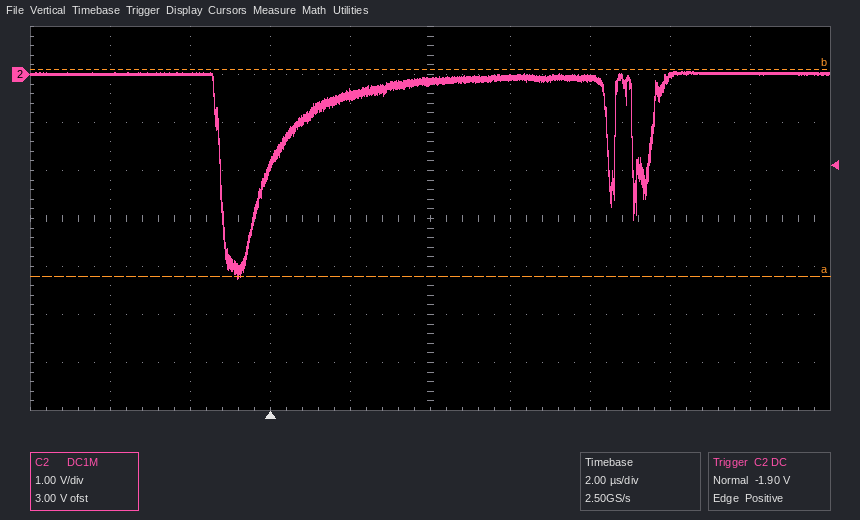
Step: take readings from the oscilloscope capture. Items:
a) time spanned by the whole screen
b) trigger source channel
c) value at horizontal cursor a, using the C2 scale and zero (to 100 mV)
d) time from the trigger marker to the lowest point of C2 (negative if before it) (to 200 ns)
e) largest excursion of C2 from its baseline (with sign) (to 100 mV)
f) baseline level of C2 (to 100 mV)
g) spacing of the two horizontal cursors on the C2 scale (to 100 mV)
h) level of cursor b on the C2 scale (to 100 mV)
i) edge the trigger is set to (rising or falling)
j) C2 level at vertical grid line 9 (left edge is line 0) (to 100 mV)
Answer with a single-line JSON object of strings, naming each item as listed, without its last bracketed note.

{"time spanned by the whole screen": "20 µs", "trigger source channel": "C2", "value at horizontal cursor a, using the C2 scale and zero": "-4.2 V", "time from the trigger marker to the lowest point of C2 (negative if before it)": "-800 ns", "largest excursion of C2 from its baseline (with sign)": "-4.3 V", "baseline level of C2": "0.0 V", "spacing of the two horizontal cursors on the C2 scale": "4.3 V", "level of cursor b on the C2 scale": "100 mV", "edge the trigger is set to": "rising", "C2 level at vertical grid line 9 (left edge is line 0)": "0.0 V"}
